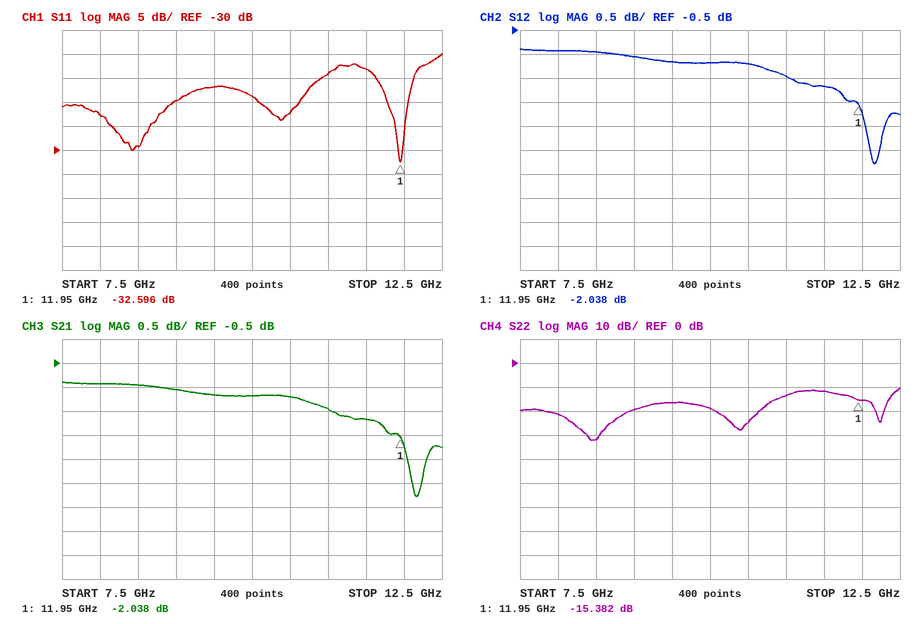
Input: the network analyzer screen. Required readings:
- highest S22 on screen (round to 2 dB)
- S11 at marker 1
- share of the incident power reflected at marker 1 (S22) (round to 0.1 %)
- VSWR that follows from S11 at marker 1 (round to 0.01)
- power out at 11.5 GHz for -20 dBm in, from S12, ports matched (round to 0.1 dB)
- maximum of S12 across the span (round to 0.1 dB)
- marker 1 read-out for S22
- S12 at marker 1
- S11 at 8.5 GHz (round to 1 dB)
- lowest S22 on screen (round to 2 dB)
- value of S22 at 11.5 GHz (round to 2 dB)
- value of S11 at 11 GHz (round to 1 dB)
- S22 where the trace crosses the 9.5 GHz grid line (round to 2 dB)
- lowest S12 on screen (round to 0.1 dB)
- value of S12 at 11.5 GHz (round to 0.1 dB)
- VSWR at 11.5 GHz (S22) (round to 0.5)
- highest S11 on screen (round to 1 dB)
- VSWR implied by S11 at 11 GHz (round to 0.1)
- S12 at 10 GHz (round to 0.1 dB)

-10 dB
-32.596 dB
2.9 %
1.05
-21.7 dBm
-0.9 dB
-15.382 dB
-2.038 dB
-29 dB
-32 dB
-12 dB
-14 dB
-16 dB
-3.3 dB
-1.7 dB
1.5
-10 dB
1.5
-1.2 dB
